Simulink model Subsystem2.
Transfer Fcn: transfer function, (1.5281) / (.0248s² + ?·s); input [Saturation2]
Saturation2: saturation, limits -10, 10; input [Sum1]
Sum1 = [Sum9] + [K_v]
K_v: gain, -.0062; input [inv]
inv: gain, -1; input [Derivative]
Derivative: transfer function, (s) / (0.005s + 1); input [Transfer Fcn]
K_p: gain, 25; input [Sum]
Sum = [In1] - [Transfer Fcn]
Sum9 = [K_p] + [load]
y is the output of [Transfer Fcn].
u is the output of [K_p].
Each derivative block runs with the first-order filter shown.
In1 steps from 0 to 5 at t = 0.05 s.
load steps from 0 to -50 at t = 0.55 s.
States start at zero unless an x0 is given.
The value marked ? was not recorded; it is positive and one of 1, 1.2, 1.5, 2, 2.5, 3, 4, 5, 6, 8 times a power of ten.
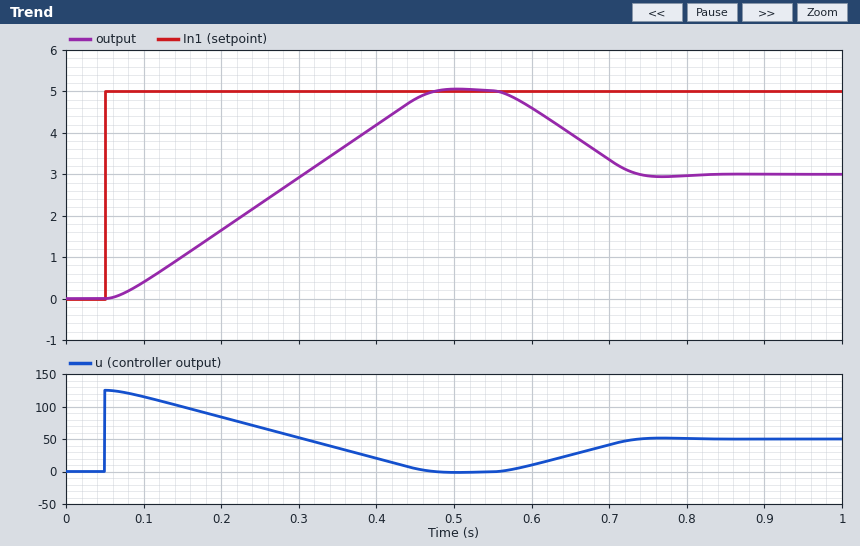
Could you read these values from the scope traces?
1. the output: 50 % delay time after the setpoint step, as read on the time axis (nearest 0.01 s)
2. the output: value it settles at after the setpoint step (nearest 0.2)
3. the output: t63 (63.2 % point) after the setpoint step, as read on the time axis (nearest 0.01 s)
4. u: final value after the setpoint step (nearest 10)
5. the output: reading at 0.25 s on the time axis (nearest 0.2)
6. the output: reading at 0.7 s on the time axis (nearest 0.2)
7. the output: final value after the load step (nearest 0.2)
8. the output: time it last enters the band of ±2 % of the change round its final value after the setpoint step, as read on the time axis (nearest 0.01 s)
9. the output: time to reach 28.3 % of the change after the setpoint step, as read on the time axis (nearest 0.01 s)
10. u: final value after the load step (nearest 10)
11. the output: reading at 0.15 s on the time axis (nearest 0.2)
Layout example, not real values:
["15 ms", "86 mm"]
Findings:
["0.27 s", "5.0", "0.32 s", "0", "2.2", "3.4", "3.0", "0.46 s", "0.18 s", "50", "1.0"]
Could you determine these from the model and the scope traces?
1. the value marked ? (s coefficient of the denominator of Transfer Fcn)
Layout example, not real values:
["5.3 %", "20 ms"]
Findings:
["1.2"]
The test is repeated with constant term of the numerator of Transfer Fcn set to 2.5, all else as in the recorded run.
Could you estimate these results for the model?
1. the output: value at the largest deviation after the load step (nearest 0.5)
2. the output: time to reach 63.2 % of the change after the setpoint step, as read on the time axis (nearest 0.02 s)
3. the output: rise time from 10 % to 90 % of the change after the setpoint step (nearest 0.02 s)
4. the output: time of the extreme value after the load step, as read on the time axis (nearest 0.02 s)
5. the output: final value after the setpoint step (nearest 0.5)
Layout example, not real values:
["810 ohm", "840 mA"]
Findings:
["3.0", "0.22 s", "0.20 s", "0.70 s", "5.0"]
